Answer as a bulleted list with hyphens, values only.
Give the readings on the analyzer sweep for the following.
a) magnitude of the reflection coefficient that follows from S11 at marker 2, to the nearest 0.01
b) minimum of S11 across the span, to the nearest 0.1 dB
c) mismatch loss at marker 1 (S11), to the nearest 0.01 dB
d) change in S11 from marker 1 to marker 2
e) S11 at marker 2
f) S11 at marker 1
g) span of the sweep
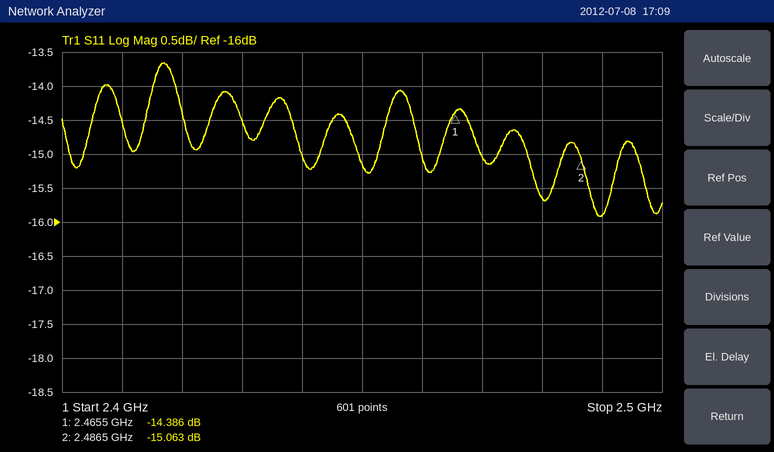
- 0.18
- -15.9 dB
- 0.16 dB
- -0.677 dB
- -15.063 dB
- -14.386 dB
- 100 MHz
